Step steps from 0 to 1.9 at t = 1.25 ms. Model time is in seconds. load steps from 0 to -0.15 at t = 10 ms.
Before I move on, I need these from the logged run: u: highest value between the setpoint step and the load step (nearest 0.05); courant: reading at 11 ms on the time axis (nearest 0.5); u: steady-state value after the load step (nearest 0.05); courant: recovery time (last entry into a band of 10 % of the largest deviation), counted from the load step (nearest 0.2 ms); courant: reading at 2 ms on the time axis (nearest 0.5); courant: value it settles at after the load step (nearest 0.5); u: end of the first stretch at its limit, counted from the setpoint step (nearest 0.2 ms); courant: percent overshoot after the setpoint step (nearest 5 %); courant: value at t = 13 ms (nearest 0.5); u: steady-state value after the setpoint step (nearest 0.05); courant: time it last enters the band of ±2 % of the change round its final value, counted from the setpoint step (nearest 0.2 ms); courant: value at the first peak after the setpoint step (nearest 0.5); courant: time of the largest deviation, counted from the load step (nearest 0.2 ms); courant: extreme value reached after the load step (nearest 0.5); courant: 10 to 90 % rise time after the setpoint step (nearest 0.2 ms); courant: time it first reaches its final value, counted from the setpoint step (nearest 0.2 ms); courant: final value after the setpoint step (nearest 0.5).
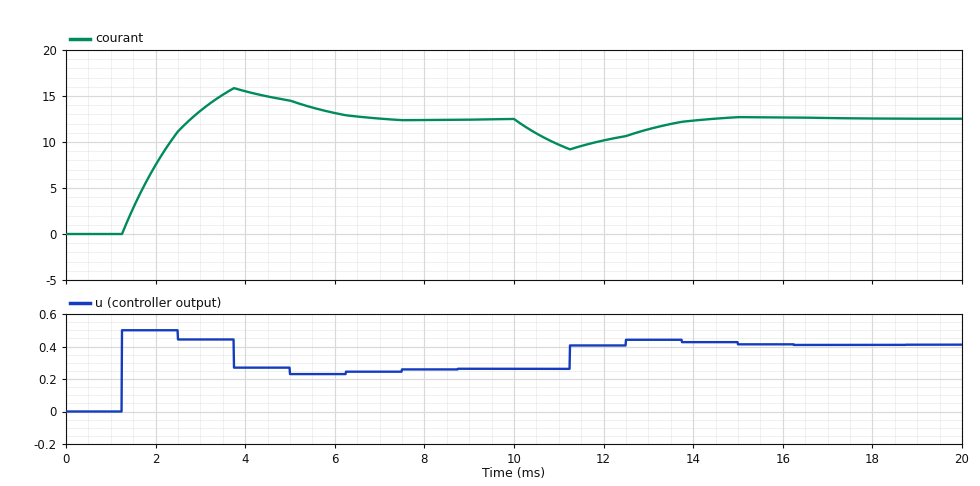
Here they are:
0.50
9.5
0.40
3.8 ms
7.5
12.5
1.2 ms
25 %
11.5
0.25
5.2 ms
16.0
1.2 ms
9.0
1.2 ms
1.6 ms
12.5
